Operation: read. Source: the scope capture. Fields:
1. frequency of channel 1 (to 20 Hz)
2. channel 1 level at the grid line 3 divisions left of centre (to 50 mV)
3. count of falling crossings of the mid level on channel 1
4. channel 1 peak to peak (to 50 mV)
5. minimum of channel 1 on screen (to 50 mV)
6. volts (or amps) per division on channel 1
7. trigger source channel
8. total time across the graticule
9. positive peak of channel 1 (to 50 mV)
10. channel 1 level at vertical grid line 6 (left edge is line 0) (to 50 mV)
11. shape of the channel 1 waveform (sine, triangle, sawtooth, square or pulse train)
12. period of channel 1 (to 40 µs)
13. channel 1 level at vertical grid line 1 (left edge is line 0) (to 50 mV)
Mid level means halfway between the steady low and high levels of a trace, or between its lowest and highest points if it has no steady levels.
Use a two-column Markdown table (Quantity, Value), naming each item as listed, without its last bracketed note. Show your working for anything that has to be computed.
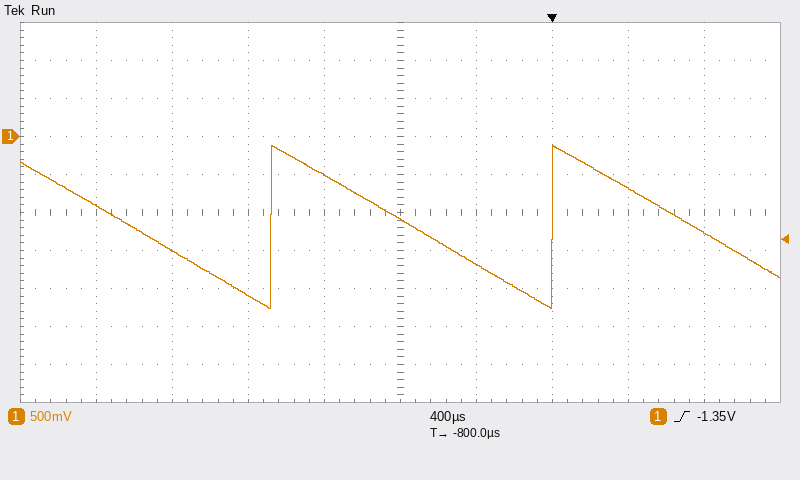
| Quantity | Value |
|---|---|
| frequency of channel 1 | 1 / 1.48 ms ≈ 676 Hz, so 680 Hz to the nearest 20 Hz |
| channel 1 level at the grid line 3 divisions left of centre | -1.50 V |
| count of falling crossings of the mid level on channel 1 | 3 |
| channel 1 peak to peak | -100 mV − (-2.25 V) = 2.15 V |
| minimum of channel 1 on screen | -2.25 V |
| volts (or amps) per division on channel 1 | 500 mV |
| trigger source channel | channel 1 |
| total time across the graticule | 4 ms |
| positive peak of channel 1 | -100 mV |
| channel 1 level at vertical grid line 6 (left edge is line 0) | -1.70 V |
| shape of the channel 1 waveform | sawtooth |
| period of channel 1 | 1.48 ms |
| channel 1 level at vertical grid line 1 (left edge is line 0) | -900 mV |
